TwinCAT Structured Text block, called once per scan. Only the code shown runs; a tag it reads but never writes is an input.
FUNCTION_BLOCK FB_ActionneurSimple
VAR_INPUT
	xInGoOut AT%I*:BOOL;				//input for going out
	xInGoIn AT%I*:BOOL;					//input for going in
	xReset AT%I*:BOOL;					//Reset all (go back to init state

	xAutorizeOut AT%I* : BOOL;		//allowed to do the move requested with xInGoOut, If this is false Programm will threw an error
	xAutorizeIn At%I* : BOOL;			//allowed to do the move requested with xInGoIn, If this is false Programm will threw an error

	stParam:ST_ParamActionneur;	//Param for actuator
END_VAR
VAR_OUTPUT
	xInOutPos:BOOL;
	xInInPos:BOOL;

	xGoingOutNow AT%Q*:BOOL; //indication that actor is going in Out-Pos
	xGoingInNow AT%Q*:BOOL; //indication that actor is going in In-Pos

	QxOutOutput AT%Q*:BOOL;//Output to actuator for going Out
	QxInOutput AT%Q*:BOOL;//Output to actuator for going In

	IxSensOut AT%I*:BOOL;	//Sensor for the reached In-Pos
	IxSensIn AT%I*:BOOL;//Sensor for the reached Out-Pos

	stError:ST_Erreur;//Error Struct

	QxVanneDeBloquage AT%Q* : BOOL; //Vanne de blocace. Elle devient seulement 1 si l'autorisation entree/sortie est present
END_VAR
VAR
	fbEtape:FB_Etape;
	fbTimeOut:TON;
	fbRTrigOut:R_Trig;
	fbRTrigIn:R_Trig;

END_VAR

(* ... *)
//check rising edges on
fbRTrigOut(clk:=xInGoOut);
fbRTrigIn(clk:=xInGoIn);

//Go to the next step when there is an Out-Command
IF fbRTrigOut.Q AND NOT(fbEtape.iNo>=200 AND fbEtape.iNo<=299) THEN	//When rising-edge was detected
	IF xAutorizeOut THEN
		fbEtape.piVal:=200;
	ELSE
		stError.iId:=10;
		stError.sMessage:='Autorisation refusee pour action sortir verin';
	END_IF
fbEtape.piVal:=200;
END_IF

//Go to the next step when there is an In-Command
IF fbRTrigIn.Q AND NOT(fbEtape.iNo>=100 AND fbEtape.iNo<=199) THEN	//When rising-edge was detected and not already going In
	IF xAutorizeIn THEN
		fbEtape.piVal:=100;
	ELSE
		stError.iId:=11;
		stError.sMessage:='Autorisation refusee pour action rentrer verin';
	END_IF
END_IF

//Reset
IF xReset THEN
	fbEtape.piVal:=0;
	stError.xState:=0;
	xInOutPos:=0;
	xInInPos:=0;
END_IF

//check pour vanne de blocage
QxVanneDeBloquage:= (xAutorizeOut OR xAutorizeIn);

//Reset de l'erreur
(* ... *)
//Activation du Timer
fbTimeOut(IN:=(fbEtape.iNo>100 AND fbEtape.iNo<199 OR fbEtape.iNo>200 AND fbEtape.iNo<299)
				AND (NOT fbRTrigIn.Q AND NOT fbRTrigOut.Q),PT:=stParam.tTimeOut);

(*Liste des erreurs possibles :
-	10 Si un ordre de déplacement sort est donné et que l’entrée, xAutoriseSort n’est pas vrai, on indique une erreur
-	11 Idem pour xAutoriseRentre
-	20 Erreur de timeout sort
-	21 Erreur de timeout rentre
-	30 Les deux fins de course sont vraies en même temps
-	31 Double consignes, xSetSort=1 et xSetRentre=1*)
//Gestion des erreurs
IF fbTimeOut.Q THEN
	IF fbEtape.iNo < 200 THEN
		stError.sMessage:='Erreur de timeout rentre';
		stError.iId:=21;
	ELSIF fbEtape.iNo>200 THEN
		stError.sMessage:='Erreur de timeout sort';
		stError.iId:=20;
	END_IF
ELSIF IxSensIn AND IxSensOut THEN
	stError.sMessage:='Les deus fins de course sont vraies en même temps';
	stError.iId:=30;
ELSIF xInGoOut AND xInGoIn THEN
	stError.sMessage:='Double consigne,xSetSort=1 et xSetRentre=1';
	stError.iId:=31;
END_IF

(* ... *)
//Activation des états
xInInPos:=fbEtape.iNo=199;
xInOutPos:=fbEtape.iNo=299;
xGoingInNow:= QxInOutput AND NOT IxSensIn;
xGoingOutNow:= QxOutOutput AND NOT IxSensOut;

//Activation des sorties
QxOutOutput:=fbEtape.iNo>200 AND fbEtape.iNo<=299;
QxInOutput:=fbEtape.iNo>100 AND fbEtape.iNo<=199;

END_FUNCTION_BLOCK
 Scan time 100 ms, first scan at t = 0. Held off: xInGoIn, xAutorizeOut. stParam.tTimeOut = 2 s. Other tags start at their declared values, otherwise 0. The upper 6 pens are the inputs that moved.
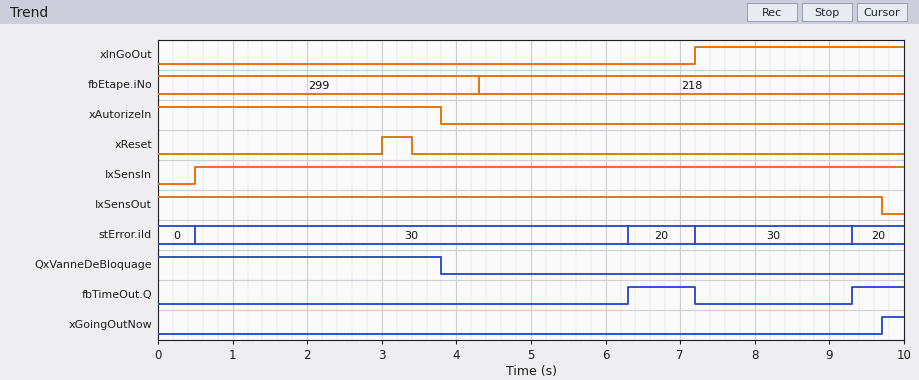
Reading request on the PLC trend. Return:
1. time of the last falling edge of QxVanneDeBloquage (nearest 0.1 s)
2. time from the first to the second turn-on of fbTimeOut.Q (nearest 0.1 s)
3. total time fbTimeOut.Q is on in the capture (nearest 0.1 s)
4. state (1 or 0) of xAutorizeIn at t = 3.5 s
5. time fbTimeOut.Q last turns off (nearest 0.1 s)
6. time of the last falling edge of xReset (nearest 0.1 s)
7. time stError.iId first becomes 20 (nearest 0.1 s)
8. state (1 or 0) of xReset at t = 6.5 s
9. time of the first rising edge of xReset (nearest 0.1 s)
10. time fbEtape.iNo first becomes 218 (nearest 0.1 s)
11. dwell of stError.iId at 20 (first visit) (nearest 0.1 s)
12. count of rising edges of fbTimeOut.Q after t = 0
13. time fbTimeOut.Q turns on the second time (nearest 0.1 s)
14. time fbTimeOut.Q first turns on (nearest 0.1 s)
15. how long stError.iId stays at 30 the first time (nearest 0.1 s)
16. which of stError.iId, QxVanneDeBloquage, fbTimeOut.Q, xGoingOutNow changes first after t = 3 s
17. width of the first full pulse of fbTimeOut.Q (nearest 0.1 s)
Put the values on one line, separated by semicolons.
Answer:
3.8 s; 3.0 s; 1.6 s; 1; 7.2 s; 3.4 s; 6.3 s; 0; 3.0 s; 4.3 s; 0.9 s; 2; 9.3 s; 6.3 s; 5.8 s; QxVanneDeBloquage; 0.9 s
